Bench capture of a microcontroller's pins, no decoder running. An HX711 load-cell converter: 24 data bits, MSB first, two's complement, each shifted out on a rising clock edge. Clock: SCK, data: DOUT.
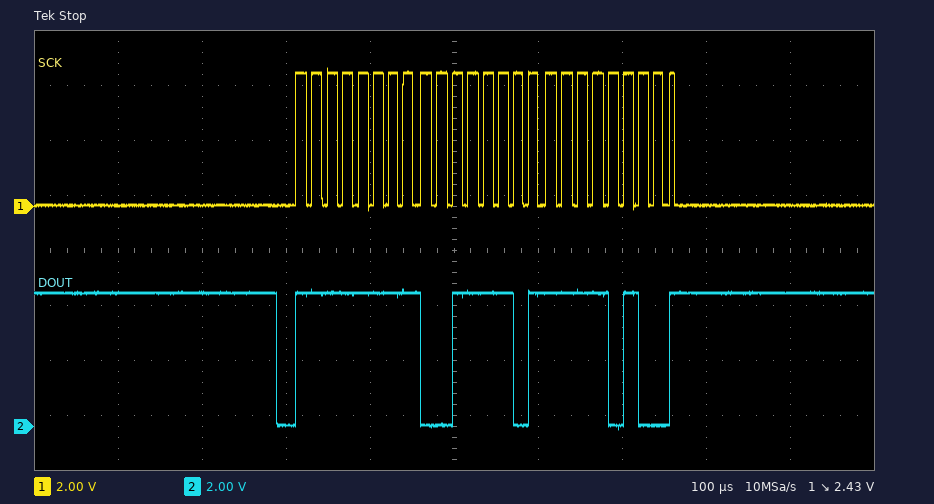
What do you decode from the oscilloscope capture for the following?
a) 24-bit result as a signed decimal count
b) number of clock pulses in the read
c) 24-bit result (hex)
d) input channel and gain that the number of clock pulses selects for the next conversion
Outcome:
-49676
25
0xFF3DF4
channel A, gain 128
